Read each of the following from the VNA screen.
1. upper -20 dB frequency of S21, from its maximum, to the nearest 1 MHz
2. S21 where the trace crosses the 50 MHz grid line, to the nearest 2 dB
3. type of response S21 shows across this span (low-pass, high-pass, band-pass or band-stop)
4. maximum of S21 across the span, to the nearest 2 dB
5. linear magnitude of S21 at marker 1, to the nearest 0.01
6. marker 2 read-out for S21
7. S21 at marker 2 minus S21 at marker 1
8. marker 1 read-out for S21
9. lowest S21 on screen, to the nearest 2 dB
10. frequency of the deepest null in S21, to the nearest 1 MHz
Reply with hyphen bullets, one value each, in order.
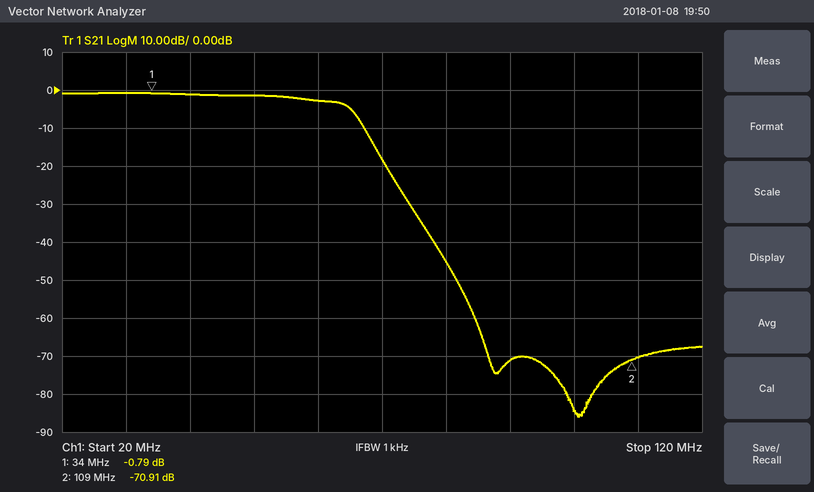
- 71 MHz
- -2 dB
- low-pass
- 0 dB
- 0.91
- -70.91 dB
- -70.12 dB
- -0.79 dB
- -86 dB
- 101 MHz
